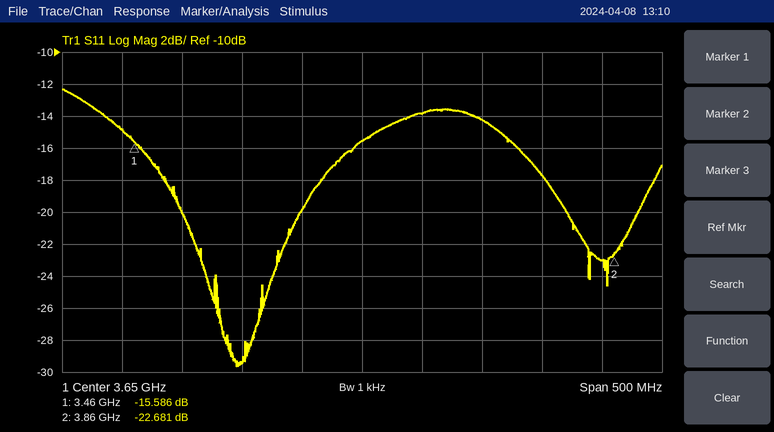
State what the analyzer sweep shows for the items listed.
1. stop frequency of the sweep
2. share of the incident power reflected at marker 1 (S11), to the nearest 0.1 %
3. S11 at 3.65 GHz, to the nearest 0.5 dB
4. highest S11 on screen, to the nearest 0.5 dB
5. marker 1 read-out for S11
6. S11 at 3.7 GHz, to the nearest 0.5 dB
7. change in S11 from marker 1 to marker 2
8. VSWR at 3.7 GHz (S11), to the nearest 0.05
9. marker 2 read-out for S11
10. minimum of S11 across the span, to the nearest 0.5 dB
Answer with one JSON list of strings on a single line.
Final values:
["3.9 GHz", "2.8 %", "-15.5 dB", "-12.5 dB", "-15.586 dB", "-14.0 dB", "-7.095 dB", "1.50", "-22.681 dB", "-29.5 dB"]
